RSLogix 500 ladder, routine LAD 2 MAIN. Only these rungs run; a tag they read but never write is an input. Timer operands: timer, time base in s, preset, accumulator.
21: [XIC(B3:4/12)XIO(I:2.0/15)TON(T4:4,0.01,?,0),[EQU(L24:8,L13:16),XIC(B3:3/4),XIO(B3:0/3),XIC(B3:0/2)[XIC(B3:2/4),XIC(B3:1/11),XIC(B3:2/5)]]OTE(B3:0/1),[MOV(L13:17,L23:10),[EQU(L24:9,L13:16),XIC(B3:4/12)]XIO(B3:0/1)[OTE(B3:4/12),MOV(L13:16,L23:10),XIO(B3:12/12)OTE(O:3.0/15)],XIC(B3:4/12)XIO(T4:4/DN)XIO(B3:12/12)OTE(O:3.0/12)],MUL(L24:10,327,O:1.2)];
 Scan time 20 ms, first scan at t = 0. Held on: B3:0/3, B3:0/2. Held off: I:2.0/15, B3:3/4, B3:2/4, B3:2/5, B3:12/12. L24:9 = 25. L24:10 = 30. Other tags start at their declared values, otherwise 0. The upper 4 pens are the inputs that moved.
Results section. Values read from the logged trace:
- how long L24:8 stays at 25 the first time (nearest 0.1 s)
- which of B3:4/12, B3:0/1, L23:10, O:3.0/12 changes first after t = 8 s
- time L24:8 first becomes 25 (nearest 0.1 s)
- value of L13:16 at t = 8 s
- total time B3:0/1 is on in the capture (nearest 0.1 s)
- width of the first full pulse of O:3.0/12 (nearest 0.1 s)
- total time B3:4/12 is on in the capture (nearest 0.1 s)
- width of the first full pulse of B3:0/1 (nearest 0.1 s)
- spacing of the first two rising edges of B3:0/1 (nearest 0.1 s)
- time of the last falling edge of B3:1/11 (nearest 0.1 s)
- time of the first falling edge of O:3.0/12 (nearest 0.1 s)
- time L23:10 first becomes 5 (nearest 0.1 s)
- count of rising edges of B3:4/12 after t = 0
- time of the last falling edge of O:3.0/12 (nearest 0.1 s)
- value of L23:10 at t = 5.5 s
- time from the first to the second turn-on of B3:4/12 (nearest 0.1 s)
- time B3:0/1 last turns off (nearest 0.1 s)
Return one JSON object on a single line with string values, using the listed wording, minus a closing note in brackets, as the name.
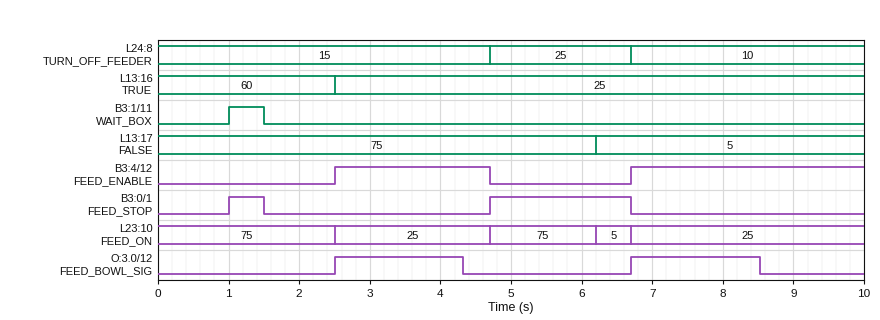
{"how long L24:8 stays at 25 the first time": "2.0 s", "which of B3:4/12, B3:0/1, L23:10, O:3.0/12 changes first after t = 8 s": "O:3.0/12", "time L24:8 first becomes 25": "4.7 s", "value of L13:16 at t = 8 s": "25", "total time B3:0/1 is on in the capture": "2.5 s", "width of the first full pulse of O:3.0/12": "1.8 s", "total time B3:4/12 is on in the capture": "5.5 s", "width of the first full pulse of B3:0/1": "0.5 s", "spacing of the first two rising edges of B3:0/1": "3.7 s", "time of the last falling edge of B3:1/11": "1.5 s", "time of the first falling edge of O:3.0/12": "4.3 s", "time L23:10 first becomes 5": "6.2 s", "count of rising edges of B3:4/12 after t = 0": "2", "time of the last falling edge of O:3.0/12": "8.5 s", "value of L23:10 at t = 5.5 s": "75", "time from the first to the second turn-on of B3:4/12": "4.2 s", "time B3:0/1 last turns off": "6.7 s"}
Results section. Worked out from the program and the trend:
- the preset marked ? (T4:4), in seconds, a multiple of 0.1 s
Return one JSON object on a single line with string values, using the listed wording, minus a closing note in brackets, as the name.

{"the preset marked ? (T4:4), in seconds, a multiple of 0.1 s": "1.8 s"}
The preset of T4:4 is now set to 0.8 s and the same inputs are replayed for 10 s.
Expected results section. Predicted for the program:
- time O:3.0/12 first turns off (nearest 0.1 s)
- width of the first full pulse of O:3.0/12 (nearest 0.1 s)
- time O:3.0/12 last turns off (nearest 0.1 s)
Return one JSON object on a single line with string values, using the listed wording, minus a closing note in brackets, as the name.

{"time O:3.0/12 first turns off": "3.3 s", "width of the first full pulse of O:3.0/12": "0.8 s", "time O:3.0/12 last turns off": "7.5 s"}
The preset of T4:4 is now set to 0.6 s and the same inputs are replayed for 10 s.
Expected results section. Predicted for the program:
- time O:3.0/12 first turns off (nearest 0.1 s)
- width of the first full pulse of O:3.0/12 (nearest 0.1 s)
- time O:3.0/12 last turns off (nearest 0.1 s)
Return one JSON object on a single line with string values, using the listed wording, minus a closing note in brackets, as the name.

{"time O:3.0/12 first turns off": "3.1 s", "width of the first full pulse of O:3.0/12": "0.6 s", "time O:3.0/12 last turns off": "7.3 s"}
